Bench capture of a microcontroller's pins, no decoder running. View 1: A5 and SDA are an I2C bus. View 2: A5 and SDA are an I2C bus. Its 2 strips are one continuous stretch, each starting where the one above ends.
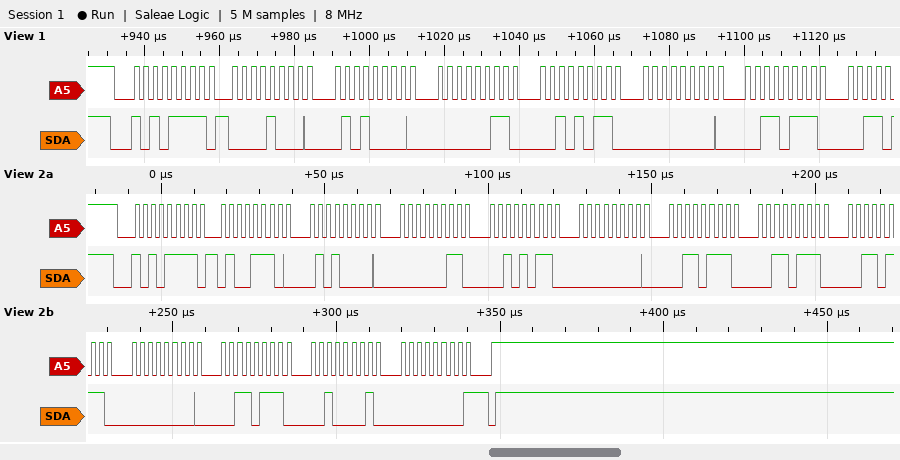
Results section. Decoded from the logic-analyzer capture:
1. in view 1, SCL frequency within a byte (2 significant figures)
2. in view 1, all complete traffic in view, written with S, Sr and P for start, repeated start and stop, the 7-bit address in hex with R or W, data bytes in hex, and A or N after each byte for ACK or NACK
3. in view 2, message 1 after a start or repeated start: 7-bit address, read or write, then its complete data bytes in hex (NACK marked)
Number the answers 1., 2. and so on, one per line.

1. 400 kHz
2. S 57R A 08 A 50 A 03 A 2B A 00 A 37 A
3. 0x57 read: 4E 50 03 2B 00 37 37 37 00 37 21 00 NACK
